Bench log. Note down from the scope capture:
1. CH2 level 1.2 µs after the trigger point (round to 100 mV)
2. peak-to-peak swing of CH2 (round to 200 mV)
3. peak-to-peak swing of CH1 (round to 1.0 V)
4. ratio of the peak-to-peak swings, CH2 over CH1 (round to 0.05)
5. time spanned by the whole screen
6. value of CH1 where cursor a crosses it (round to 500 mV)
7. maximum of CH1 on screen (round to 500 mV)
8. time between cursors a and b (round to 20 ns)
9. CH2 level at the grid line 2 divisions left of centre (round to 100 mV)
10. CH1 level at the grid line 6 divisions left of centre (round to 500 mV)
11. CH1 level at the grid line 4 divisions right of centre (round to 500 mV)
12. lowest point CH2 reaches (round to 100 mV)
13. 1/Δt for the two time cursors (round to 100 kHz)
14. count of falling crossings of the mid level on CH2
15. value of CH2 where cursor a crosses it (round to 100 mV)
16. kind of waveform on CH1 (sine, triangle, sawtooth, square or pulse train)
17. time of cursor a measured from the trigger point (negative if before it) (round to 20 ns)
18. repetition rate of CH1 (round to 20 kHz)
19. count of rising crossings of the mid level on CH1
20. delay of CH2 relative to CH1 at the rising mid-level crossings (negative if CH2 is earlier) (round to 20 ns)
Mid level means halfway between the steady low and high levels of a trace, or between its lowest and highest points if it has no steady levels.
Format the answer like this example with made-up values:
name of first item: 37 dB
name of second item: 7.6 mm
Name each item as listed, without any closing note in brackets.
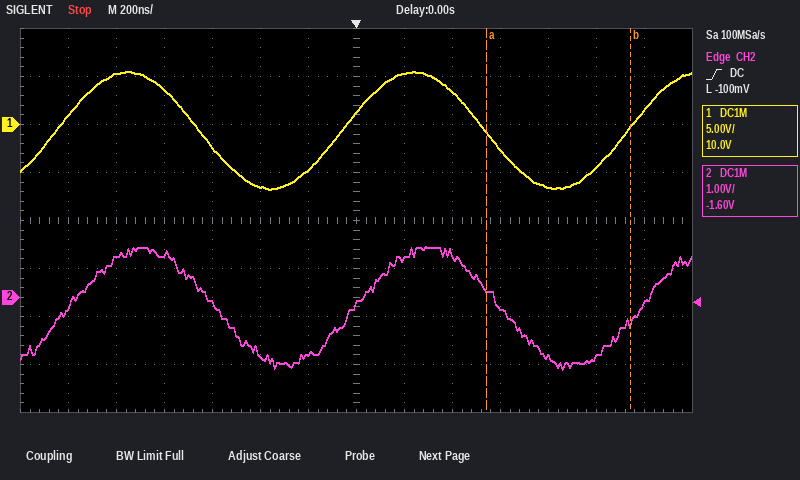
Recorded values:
CH2 level 1.2 µs after the trigger point: -100 mV
peak-to-peak swing of CH2: 2.6 V
peak-to-peak swing of CH1: 12.0 V
ratio of the peak-to-peak swings, CH2 over CH1: 0.20
time spanned by the whole screen: 2.8 µs
value of CH1 where cursor a crosses it: -1.0 V
maximum of CH1 on screen: 5.5 V
time between cursors a and b: 600 ns
CH2 level at the grid line 2 divisions left of centre: -1.2 V
CH1 level at the grid line 6 divisions left of centre: 1.0 V
CH1 level at the grid line 4 divisions right of centre: -6.5 V
lowest point CH2 reaches: -1.5 V
1/Δt for the two time cursors: 1.7 MHz
count of falling crossings of the mid level on CH2: 2
value of CH2 where cursor a crosses it: 200 mV
kind of waveform on CH1: sine
time of cursor a measured from the trigger point (negative if before it): +540 ns
repetition rate of CH1: 840 kHz
count of rising crossings of the mid level on CH1: 3
delay of CH2 relative to CH1 at the rising mid-level crossings (negative if CH2 is earlier): +60 ns
